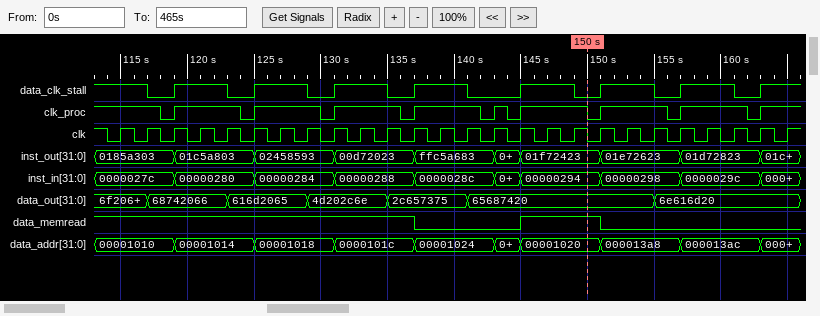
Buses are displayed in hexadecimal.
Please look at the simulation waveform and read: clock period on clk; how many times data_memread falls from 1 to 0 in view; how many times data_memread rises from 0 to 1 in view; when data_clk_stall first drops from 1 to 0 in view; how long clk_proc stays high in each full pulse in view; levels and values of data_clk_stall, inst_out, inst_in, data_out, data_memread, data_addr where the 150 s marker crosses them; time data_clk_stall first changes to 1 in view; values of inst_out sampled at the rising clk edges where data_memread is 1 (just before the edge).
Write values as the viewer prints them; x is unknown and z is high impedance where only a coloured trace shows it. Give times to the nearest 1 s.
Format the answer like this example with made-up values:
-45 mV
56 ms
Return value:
2 s
2
1
117 s
5 s, 5 s, 5 s, 5 s, 1 s, 5 s, 5 s, 5 s
data_clk_stall=0, inst_out=01f72423, inst_in=00000294, data_out=65687420, data_memread=1, data_addr=00001020
119 s
0185a303, 0185a303, 0185a303, 01c5a803, 01c5a803, 01c5a803, 02458593, 02458593, 02458593, 00d72023, 00d72023, 00d72023, 01f72423, 01f72423, 01f72423
